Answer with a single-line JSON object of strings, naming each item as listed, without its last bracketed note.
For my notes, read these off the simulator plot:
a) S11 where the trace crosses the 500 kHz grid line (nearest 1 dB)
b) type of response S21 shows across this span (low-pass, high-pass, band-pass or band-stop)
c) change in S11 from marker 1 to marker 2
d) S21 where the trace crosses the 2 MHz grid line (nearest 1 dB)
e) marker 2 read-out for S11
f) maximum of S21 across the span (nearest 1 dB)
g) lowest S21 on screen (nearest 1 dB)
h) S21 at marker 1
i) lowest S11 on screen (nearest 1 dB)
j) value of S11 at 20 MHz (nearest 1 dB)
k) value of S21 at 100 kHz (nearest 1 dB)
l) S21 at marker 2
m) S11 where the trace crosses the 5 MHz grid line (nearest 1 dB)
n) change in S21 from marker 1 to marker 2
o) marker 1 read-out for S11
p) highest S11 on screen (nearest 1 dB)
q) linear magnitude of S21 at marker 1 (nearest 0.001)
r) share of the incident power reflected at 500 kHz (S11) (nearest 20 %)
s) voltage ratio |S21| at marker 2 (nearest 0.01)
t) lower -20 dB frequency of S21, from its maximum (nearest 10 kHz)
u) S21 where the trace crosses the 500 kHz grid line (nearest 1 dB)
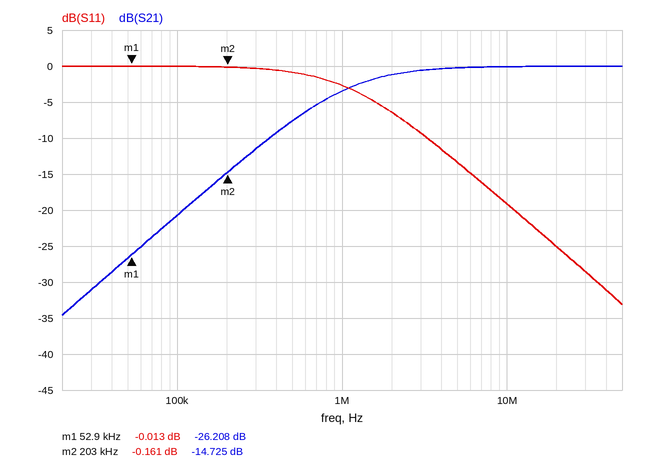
{"S11 where the trace crosses the 500 kHz grid line": "-1 dB", "type of response S21 shows across this span": "high-pass", "change in S11 from marker 1 to marker 2": "-0.148 dB", "S21 where the trace crosses the 2 MHz grid line": "-1 dB", "marker 2 read-out for S11": "-0.161 dB", "maximum of S21 across the span": "0 dB", "lowest S21 on screen": "-35 dB", "S21 at marker 1": "-26.208 dB", "lowest S11 on screen": "-33 dB", "value of S11 at 20 MHz": "-25 dB", "value of S21 at 100 kHz": "-21 dB", "S21 at marker 2": "-14.725 dB", "S11 where the trace crosses the 5 MHz grid line": "-13 dB", "change in S21 from marker 1 to marker 2": "11.483 dB", "marker 1 read-out for S11": "-0.013 dB", "highest S11 on screen": "0 dB", "linear magnitude of S21 at marker 1": "0.049", "share of the incident power reflected at 500 kHz (S11)": "80 %", "voltage ratio |S21| at marker 2": "0.18", "lower -20 dB frequency of S21, from its maximum": "110 kHz", "S21 where the trace crosses the 500 kHz grid line": "-8 dB"}
